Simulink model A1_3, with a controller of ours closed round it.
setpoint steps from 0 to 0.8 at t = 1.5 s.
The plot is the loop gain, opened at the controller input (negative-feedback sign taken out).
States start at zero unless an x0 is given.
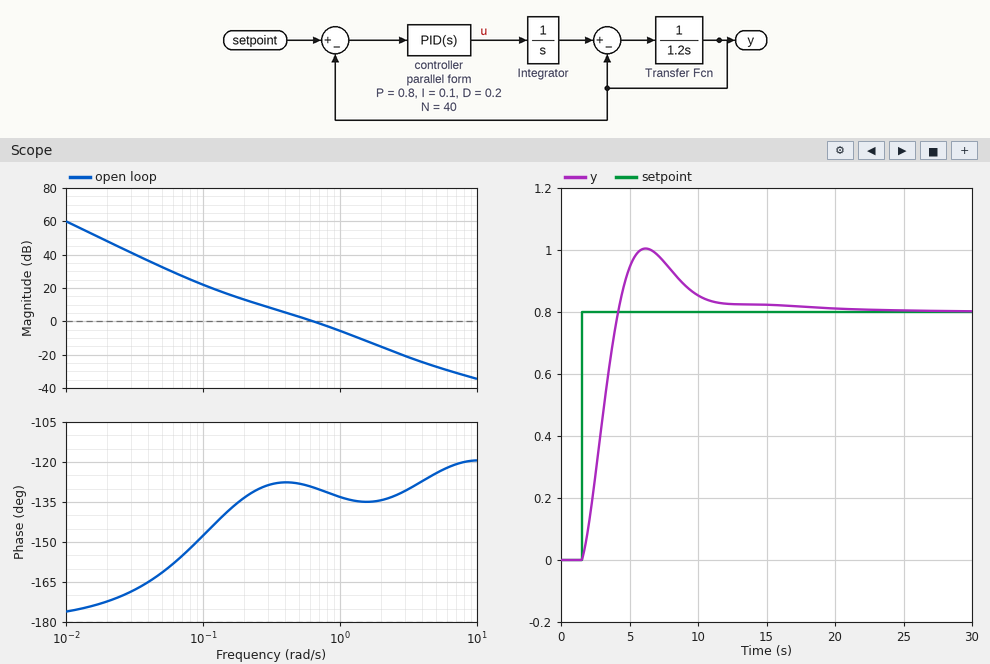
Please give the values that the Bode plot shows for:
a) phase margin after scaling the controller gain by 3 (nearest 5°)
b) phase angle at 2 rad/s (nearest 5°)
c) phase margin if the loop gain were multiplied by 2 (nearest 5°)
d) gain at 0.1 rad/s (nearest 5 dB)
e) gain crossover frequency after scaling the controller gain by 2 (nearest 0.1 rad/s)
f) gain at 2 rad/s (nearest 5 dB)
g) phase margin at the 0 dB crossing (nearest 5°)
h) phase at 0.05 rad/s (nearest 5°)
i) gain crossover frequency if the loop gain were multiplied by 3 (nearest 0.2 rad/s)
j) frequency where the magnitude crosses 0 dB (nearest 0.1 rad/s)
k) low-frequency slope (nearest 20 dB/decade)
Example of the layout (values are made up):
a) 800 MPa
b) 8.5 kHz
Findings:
a) 45°
b) -135°
c) 45°
d) 20 dB
e) 1.0 rad/s
f) -15 dB
g) 50°
h) -160°
i) 1.4 rad/s
j) 0.6 rad/s
k) -40 dB/decade
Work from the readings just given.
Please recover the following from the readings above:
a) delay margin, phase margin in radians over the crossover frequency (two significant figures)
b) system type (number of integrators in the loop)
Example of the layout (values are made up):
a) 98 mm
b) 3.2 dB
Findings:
a) 1.5 s
b) 2
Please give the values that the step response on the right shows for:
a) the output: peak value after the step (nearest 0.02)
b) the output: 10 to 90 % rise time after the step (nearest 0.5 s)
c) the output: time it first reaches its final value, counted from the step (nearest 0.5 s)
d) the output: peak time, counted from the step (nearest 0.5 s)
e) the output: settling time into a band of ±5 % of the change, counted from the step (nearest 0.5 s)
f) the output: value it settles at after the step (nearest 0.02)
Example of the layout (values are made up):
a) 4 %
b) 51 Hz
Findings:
a) 1.00
b) 2.0 s
c) 2.5 s
d) 4.5 s
e) 9.0 s
f) 0.80
